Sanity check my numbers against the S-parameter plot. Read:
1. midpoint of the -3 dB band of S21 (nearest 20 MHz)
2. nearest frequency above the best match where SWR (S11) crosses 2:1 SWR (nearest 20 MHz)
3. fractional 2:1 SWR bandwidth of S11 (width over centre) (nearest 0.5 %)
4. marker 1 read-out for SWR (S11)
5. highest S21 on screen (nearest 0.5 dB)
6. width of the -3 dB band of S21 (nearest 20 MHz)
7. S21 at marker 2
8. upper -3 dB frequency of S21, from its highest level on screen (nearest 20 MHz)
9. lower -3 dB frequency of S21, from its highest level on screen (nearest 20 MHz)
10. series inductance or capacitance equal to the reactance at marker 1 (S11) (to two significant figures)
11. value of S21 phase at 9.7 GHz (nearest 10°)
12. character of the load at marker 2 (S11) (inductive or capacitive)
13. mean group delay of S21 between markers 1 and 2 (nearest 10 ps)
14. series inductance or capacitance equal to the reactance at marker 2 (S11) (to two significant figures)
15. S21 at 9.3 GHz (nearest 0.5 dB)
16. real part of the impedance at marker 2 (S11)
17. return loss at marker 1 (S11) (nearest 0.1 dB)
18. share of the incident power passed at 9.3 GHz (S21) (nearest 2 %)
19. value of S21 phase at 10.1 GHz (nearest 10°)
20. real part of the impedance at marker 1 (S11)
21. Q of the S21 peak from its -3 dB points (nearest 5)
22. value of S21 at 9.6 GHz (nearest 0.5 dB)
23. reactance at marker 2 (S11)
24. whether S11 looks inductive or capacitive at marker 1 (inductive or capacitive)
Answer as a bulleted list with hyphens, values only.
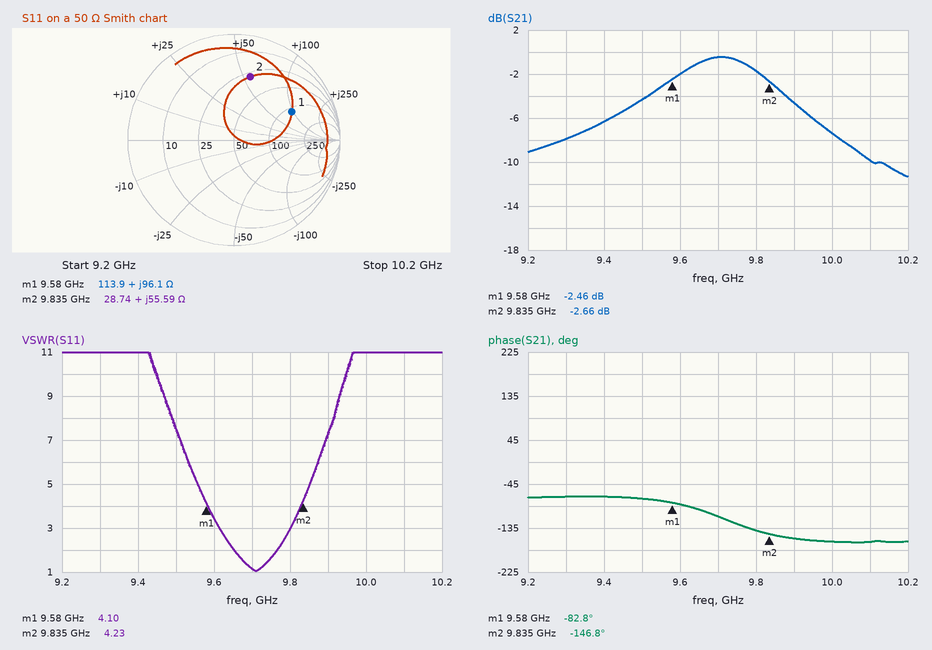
- 9.70 GHz
- 9.76 GHz
- 1.0 %
- 4.10
- -0.5 dB
- 320 MHz
- -2.66 dB
- 9.86 GHz
- 9.54 GHz
- 1.6 nH
- -110°
- inductive
- 700 ps
- 900 pH
- -8.0 dB
- 28.74 Ω
- 4.3 dB
- 16 %
- -160°
- 113.9 Ω
- 30
- -2.0 dB
- +55.59 Ω
- inductive
